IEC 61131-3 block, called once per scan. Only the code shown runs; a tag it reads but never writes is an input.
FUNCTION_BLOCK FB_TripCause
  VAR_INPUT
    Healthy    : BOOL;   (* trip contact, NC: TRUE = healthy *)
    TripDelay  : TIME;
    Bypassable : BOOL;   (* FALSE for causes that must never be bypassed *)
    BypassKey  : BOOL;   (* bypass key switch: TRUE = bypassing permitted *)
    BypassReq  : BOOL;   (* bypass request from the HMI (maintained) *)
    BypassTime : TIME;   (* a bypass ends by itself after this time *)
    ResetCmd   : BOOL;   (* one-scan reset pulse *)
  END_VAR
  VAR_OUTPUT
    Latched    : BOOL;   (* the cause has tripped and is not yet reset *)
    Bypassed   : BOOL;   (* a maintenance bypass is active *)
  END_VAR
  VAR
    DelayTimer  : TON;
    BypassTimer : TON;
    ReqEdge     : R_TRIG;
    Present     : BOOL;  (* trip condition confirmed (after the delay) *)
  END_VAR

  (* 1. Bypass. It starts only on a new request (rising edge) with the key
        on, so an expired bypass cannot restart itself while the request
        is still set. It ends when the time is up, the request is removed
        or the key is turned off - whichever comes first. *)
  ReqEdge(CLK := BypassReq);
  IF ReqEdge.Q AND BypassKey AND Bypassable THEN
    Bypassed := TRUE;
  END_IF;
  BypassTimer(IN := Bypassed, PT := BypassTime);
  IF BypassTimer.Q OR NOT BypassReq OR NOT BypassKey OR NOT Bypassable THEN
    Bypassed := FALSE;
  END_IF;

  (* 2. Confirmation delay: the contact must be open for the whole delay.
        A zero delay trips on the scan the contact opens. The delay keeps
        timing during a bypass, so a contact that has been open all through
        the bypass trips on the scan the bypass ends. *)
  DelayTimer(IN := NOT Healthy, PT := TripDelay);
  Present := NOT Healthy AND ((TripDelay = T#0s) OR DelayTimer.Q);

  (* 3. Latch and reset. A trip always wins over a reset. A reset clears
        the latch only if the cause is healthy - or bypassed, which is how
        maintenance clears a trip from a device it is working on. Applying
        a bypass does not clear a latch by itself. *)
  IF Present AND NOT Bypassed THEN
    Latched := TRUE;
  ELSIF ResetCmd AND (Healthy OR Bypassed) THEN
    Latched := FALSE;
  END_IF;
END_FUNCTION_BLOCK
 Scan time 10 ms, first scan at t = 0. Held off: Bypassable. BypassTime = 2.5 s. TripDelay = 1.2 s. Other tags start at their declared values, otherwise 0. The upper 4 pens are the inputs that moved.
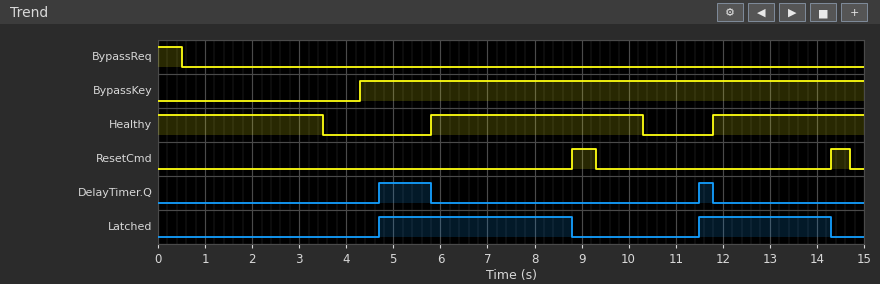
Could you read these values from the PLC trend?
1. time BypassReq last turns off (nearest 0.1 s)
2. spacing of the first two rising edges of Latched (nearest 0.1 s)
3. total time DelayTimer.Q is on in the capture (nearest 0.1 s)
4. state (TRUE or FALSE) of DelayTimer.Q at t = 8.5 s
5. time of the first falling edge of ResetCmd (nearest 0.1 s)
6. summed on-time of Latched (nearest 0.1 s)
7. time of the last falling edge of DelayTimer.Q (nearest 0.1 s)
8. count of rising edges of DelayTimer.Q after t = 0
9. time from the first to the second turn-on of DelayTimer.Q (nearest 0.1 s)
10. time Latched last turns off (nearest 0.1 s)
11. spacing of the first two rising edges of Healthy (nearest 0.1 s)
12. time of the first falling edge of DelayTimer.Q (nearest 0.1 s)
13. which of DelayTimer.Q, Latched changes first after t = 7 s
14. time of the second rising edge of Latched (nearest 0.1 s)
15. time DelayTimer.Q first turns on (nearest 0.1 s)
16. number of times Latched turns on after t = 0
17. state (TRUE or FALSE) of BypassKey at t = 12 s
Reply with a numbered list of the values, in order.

1. 0.5 s
2. 6.8 s
3. 1.4 s
4. FALSE
5. 9.3 s
6. 6.9 s
7. 11.8 s
8. 2
9. 6.8 s
10. 14.3 s
11. 6.0 s
12. 5.8 s
13. Latched
14. 11.5 s
15. 4.7 s
16. 2
17. TRUE
